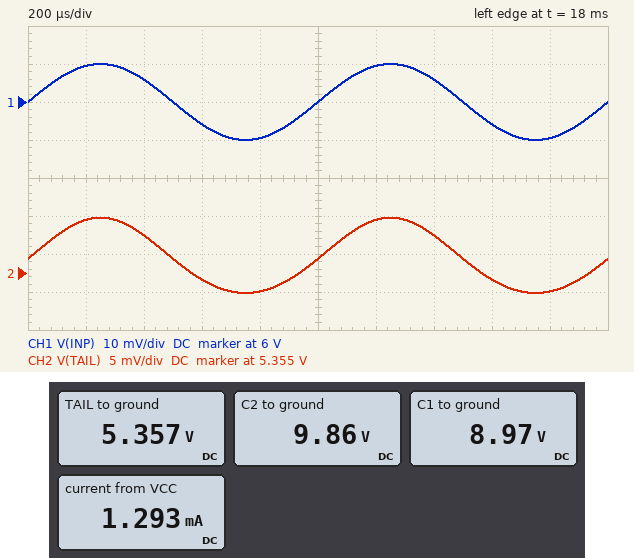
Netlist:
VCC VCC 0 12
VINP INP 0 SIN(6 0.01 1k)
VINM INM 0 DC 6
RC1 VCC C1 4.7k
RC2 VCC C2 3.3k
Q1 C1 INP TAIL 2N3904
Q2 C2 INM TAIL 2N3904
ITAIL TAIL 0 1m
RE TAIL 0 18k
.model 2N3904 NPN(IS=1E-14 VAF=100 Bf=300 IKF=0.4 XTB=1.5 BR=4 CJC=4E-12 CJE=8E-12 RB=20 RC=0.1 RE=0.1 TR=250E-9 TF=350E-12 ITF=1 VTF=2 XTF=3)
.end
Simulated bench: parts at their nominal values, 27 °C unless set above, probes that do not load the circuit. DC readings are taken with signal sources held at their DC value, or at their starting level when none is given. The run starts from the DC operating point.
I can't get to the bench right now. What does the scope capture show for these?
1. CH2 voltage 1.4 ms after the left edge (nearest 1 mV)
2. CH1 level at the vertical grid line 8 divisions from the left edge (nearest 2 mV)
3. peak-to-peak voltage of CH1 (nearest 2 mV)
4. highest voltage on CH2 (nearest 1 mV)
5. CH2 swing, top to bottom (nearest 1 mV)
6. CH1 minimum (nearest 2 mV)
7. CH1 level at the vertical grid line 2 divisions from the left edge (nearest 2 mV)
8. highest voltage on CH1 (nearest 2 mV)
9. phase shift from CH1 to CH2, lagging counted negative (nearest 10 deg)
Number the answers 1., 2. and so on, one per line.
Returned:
1. 5.360 V
2. 5.994 V
3. 20 mV
4. 5.362 V
5. 10 mV
6. 5.990 V
7. 6.006 V
8. 6.010 V
9. 0 deg
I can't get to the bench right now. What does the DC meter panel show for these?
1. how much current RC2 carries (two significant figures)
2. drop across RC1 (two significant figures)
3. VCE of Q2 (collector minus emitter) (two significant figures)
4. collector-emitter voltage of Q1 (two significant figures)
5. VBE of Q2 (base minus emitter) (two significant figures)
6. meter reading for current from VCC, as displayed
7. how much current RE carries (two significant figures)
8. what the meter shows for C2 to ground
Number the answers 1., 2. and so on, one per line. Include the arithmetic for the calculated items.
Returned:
1. (12 V - 9.86 V) / 3.3 kΩ = 650 µA
2. 12 V - 8.97 V = 3.0 V
3. 9.86 V - 5.357 V = 4.5 V
4. 8.97 V - 5.357 V = 3.6 V
5. 6 V - 5.357 V = 640 mV
6. 1.293 mA
7. (5.357 V) / 18 kΩ = 300 µA
8. 9.86 V
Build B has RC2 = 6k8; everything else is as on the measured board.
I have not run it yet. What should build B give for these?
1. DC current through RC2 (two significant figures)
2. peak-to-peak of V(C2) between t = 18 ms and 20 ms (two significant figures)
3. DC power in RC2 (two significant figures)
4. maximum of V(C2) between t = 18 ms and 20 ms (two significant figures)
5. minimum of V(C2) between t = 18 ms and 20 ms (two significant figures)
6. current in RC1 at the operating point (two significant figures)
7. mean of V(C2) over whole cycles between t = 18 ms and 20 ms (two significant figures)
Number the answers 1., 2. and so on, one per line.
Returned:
1. 640 µA
2. 1.6 V
3. 2.8 mW
4. 8.4 V
5. 6.8 V
6. 650 µA
7. 7.6 V
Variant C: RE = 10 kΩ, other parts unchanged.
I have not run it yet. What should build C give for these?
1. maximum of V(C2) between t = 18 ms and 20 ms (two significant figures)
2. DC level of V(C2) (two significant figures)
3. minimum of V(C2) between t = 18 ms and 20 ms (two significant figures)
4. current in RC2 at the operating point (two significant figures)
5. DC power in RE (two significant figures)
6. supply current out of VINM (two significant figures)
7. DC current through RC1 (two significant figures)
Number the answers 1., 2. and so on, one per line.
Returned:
1. 9.9 V
2. 9.5 V
3. 9.0 V
4. 770 µA
5. 2.9 mW
6. 2.5 µA
7. 760 µA
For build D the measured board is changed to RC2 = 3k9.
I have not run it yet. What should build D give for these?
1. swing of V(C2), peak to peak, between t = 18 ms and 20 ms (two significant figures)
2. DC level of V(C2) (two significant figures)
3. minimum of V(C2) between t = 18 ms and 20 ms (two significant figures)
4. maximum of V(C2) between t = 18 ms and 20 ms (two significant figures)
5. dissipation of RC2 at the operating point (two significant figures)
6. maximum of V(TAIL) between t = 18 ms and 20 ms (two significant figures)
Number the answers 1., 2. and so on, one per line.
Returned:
1. 930 mV
2. 9.5 V
3. 9.0 V
4. 9.9 V
5. 1.6 mW
6. 5.4 V
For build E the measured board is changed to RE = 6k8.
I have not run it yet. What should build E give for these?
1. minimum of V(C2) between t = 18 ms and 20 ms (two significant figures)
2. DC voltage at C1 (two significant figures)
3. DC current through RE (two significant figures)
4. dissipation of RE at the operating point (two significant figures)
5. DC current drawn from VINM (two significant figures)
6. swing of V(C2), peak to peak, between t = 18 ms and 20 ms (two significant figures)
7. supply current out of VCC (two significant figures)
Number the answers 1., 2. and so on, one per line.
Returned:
1. 8.5 V
2. 7.8 V
3. 790 µA
4. 4.2 mW
5. 2.9 µA
6. 1.1 V
7. 1.8 mA
